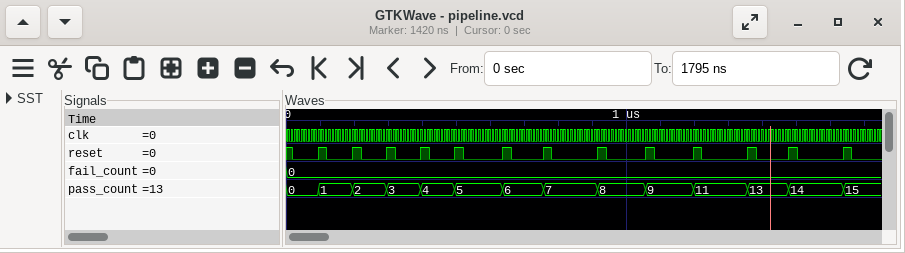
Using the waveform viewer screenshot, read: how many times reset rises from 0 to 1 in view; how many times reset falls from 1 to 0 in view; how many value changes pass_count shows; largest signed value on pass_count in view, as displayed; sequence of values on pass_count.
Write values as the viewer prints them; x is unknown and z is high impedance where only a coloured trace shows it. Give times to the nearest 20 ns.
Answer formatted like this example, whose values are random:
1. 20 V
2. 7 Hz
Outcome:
1. 13
2. 14
3. 13
4. 15
5. 0, 1, 2, 3, 4, 5, 6, 7, 8, 9, 11, 13, 14, 15
